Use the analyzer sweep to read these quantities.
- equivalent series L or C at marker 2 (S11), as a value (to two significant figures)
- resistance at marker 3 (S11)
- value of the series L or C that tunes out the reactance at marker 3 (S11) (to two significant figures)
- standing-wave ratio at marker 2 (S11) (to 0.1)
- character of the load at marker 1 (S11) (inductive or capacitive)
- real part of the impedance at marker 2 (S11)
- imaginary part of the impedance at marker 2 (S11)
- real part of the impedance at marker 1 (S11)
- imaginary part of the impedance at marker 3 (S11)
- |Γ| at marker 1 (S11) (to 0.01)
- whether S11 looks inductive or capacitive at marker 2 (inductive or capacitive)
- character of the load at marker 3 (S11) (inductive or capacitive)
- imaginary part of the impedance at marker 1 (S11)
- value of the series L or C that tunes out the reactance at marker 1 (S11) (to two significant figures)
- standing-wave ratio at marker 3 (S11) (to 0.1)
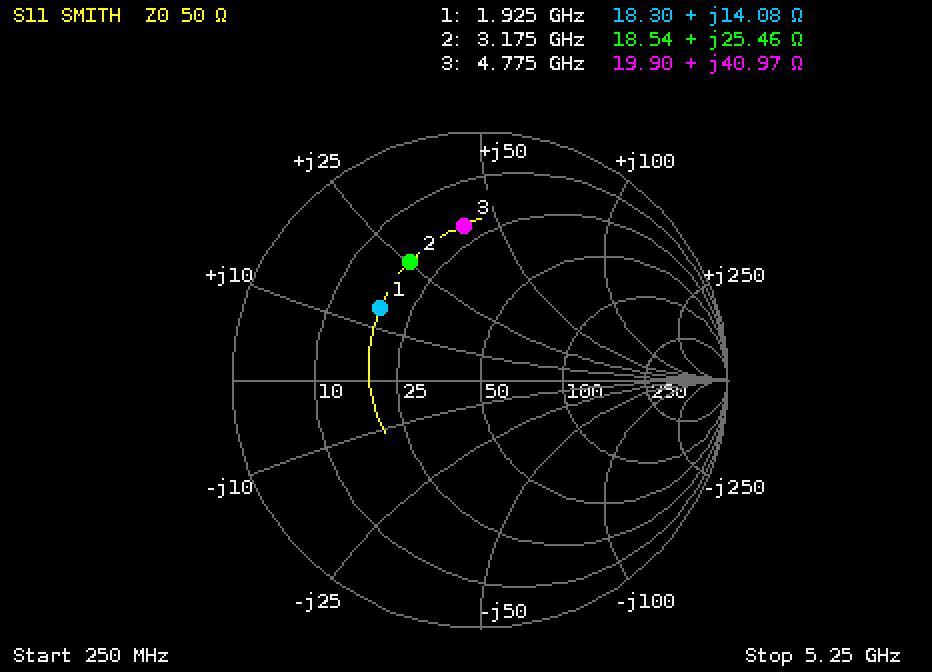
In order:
1.3 nH
19.90 Ω
810 fF
3.5
inductive
18.54 Ω
+25.46 Ω
18.30 Ω
+40.97 Ω
0.50
inductive
inductive
+14.08 Ω
5.9 pF
4.4
